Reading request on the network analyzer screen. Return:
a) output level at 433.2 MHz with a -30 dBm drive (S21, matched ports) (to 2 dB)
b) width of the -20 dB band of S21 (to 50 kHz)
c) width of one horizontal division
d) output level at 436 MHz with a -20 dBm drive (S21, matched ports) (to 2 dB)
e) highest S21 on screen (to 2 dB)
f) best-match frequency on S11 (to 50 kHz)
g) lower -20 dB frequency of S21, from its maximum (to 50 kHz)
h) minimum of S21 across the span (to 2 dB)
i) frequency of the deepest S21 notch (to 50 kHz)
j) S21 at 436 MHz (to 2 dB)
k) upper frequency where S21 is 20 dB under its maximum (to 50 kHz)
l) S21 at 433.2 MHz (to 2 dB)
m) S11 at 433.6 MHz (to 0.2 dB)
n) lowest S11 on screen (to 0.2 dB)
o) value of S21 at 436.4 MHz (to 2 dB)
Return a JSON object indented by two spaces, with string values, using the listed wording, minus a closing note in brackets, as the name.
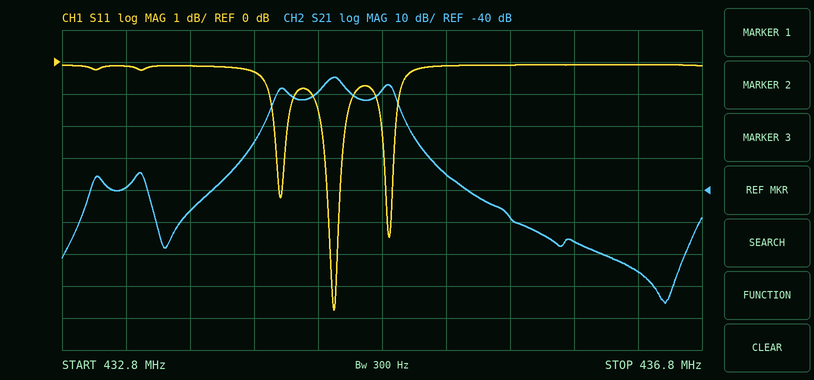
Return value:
{
  "output level at 433.2 MHz with a -30 dBm drive (S21, matched ports)": "-70 dBm",
  "width of the -20 dB band of S21": "1.00 MHz",
  "width of one horizontal division": "400 kHz",
  "output level at 436 MHz with a -20 dBm drive (S21, matched ports)": "-76 dBm",
  "highest S21 on screen": "-4 dB",
  "best-match frequency on S11": "434.50 MHz",
  "lower -20 dB frequency of S21, from its maximum": "434.00 MHz",
  "minimum of S21 across the span": "-76 dB",
  "frequency of the deepest S21 notch": "436.55 MHz",
  "S21 at 436 MHz": "-56 dB",
  "upper frequency where S21 is 20 dB under its maximum": "435.00 MHz",
  "S21 at 433.2 MHz": "-40 dB",
  "S11 at 433.6 MHz": "-0.2 dB",
  "lowest S11 on screen": "-7.8 dB",
  "value of S21 at 436.4 MHz": "-66 dB"
}
